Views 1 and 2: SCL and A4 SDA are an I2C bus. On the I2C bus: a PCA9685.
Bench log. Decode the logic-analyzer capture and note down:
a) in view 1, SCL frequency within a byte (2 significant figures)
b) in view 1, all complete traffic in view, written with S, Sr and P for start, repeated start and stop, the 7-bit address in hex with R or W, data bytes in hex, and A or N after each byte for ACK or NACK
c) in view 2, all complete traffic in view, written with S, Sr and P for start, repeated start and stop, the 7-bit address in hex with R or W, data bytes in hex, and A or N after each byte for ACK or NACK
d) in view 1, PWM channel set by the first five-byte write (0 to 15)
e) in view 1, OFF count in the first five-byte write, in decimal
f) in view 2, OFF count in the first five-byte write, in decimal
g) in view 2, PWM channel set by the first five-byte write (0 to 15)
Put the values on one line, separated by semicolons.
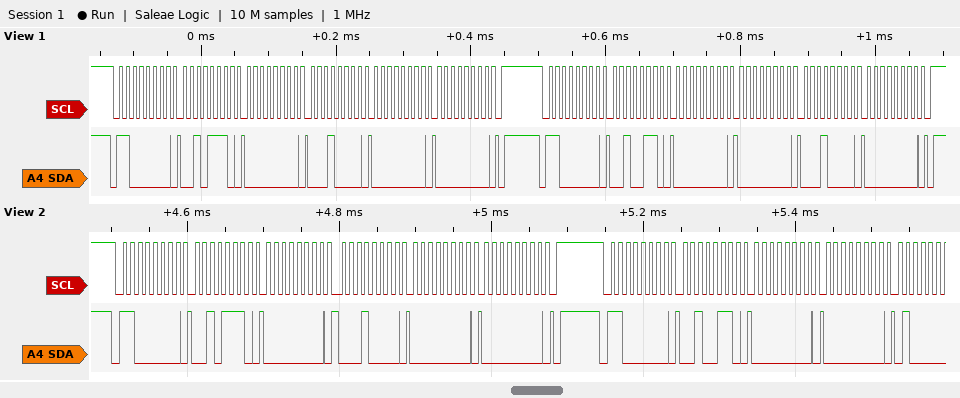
100 kHz; S 60W A 2E A 00 A 10 A 00 A 00 A P S 60W A 26 A 00 A 00 A 10 A 00 A P; S 60W A 2E A 00 A 10 A 00 A 00 A P S 60W A 26 A 00 A 00 A; 10; 0; 0; 10
